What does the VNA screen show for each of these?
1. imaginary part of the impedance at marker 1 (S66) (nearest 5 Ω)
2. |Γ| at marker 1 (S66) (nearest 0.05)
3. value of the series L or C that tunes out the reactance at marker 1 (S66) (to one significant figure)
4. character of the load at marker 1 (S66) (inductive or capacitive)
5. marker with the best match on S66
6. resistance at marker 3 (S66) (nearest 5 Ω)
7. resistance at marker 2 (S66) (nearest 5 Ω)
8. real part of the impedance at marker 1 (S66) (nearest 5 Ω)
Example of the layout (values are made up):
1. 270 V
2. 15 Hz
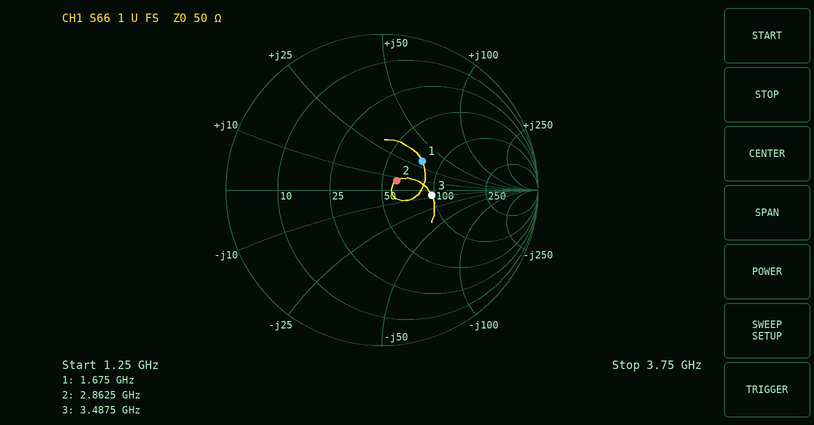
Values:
1. +30 Ω
2. 0.30
3. 3 pF
4. inductive
5. marker 2
6. 95 Ω
7. 60 Ω
8. 75 Ω
